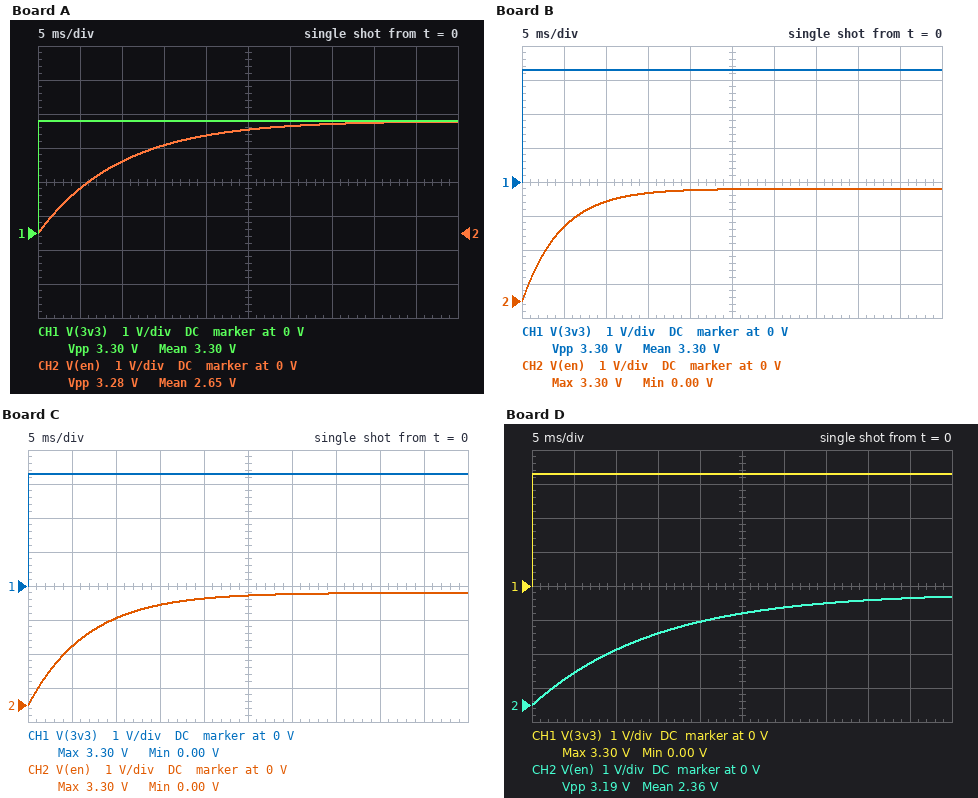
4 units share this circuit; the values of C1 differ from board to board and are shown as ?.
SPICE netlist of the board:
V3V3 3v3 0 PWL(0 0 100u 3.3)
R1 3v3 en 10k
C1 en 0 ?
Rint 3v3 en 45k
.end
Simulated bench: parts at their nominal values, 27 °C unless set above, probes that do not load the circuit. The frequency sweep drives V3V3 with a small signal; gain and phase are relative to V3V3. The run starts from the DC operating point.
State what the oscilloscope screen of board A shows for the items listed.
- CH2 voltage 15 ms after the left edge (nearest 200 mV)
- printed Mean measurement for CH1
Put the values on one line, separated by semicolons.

2.6 V; 3.30 V
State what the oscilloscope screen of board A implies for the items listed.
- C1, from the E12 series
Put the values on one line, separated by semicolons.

1.2 µF
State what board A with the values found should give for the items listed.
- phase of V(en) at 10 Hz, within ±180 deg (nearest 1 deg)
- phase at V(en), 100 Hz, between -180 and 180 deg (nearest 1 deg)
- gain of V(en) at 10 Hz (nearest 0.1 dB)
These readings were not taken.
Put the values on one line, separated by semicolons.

-32 deg; -81 deg; -1.4 dB
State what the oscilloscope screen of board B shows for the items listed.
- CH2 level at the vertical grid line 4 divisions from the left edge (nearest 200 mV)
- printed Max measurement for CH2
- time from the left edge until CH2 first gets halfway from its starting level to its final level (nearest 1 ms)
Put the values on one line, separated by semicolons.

3.2 V; 3.30 V; 3 ms
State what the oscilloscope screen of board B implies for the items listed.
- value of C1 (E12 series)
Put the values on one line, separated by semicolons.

560 nF
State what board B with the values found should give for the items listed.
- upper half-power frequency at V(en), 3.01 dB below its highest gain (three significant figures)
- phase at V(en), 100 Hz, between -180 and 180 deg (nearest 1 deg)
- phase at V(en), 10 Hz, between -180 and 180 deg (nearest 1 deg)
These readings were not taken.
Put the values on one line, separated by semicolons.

34.7 Hz; -71 deg; -16 deg
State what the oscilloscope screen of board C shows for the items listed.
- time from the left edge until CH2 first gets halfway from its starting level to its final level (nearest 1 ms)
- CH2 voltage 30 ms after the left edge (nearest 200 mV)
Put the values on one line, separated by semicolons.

5 ms; 3.2 V
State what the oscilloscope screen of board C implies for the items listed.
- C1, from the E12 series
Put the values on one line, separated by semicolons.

820 nF
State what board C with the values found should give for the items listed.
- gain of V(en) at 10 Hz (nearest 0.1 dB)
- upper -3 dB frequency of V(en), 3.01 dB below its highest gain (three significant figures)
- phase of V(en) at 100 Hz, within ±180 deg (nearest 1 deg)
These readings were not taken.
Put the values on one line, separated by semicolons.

-0.7 dB; 23.7 Hz; -77 deg
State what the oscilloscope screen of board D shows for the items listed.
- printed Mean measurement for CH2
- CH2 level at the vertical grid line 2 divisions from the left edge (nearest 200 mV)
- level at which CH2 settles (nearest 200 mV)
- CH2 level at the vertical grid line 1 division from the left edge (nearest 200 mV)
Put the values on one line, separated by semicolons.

2.36 V; 1.6 V; 3.2 V; 1.0 V
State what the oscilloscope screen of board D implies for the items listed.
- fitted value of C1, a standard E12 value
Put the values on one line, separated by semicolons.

1.8 µF
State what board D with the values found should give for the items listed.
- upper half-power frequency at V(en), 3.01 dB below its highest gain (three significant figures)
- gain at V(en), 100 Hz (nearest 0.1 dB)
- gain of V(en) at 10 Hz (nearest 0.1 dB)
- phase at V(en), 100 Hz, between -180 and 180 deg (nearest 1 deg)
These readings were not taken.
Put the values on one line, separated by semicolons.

10.8 Hz; -19.4 dB; -2.7 dB; -84 deg
